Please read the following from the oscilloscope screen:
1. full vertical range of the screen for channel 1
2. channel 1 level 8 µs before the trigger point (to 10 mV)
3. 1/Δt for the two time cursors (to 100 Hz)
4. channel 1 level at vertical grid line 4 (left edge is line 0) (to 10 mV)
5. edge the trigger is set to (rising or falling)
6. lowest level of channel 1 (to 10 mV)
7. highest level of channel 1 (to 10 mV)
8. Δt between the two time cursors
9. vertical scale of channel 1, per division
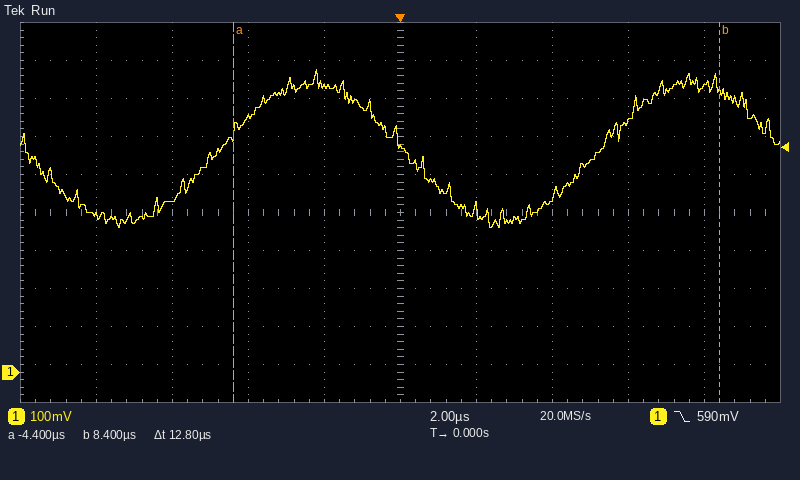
1 V
410 mV
78.1 kHz
760 mV
falling
380 mV
800 mV
12.8 µs
100 mV
